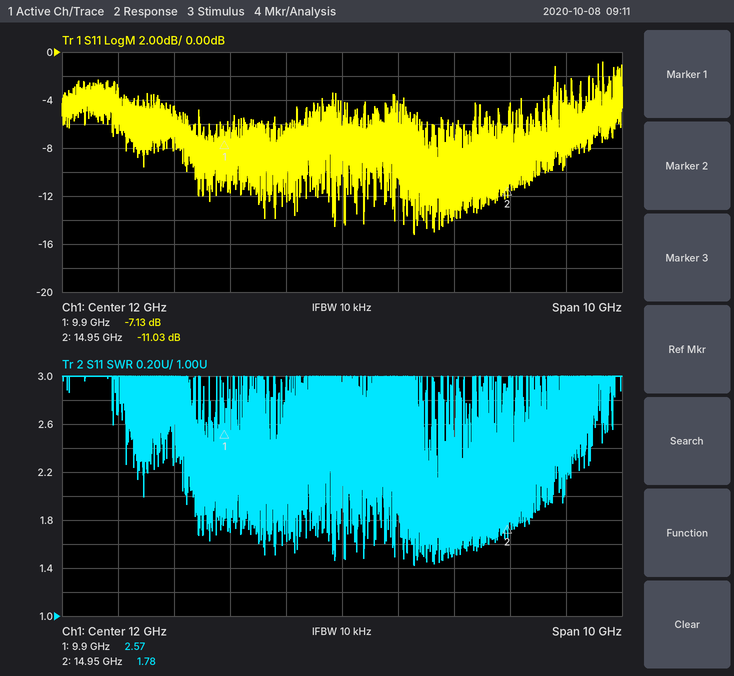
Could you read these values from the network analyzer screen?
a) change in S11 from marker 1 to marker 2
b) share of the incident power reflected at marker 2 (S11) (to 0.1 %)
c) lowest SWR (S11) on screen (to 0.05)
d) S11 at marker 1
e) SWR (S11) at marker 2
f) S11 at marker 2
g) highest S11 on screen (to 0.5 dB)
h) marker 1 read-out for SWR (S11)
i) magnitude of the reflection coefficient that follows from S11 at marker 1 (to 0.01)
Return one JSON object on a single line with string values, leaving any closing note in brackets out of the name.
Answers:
{"change in S11 from marker 1 to marker 2": "-3.90 dB", "share of the incident power reflected at marker 2 (S11)": "7.9 %", "lowest SWR (S11) on screen": "1.40", "S11 at marker 1": "-7.13 dB", "SWR (S11) at marker 2": "1.78", "S11 at marker 2": "-11.03 dB", "highest S11 on screen": "-1.0 dB", "marker 1 read-out for SWR": "2.57", "magnitude of the reflection coefficient that follows from S11 at marker 1": "0.44"}
